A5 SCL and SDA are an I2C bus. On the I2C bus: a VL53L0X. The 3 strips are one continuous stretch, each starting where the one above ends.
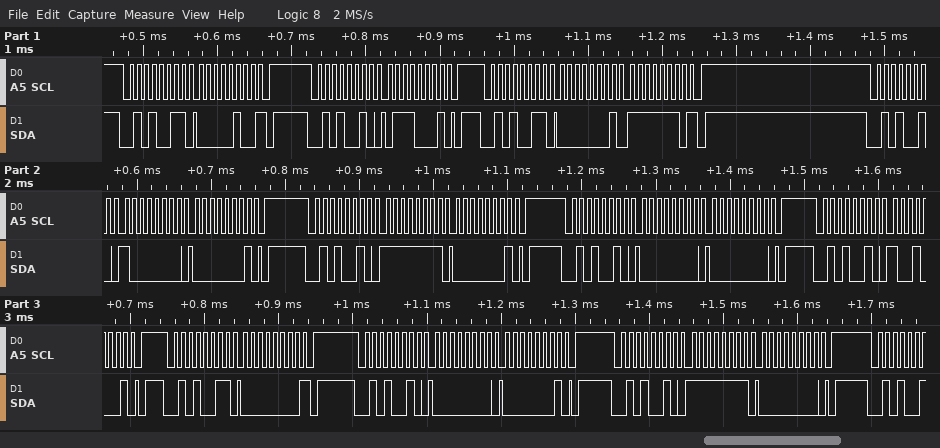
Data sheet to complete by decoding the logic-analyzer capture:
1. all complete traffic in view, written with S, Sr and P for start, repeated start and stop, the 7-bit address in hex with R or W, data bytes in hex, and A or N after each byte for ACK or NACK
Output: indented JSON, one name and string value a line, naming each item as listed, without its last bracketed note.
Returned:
{
  "all complete traffic in view, written with S, Sr and P for start, repeated start and stop, the 7-bit address in hex with R or W, data bytes in hex, and A or N after each byte for ACK or NACK": "S 29R A 04 N P S 29W A 71 A P S 29R A 01 A FE N P S 29W A 80 A 01 A P S 29W A FF A 01 A P S 29W A 00 A 00 A P S 29W A 91 A P S 29R A 00 N P S 29W A 00 A 01 A P S 29W A FF A 00 A P"
}
